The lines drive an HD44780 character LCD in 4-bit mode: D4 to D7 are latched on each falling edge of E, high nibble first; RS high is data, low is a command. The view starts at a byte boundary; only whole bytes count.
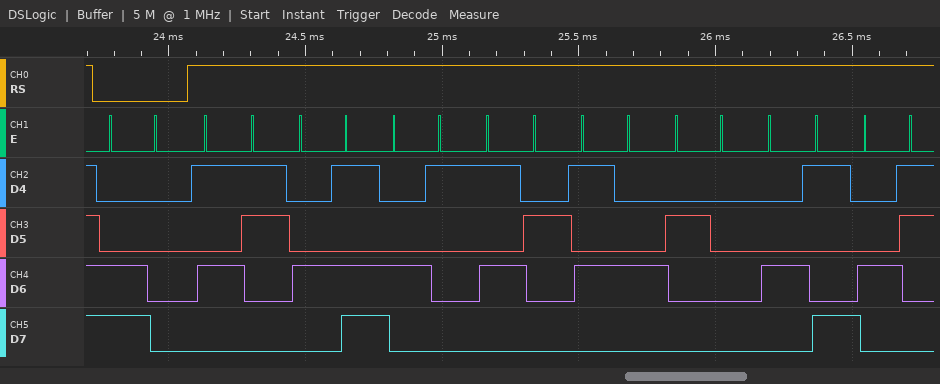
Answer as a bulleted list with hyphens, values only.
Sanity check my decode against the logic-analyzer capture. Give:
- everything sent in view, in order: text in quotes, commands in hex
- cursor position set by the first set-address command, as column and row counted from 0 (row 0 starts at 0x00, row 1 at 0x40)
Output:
- 0xC0 "SMART IC"
- column 0, row 1
